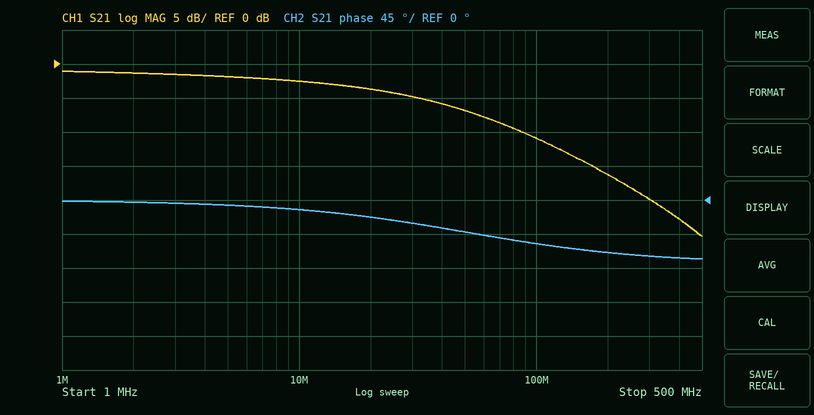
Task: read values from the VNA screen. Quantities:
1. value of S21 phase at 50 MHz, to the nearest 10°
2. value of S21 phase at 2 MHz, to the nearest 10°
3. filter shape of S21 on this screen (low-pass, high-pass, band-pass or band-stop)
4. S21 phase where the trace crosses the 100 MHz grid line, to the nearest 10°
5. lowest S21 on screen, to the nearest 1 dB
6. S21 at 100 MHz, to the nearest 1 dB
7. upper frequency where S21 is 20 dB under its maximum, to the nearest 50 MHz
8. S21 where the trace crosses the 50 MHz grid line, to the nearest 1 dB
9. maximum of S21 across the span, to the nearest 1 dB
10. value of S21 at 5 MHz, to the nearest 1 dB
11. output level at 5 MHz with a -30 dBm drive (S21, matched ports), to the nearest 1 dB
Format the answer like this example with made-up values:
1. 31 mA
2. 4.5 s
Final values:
1. -40°
2. 0°
3. low-pass
4. -60°
5. -25 dB
6. -11 dB
7. 350 MHz
8. -7 dB
9. -1 dB
10. -2 dB
11. -32 dBm
